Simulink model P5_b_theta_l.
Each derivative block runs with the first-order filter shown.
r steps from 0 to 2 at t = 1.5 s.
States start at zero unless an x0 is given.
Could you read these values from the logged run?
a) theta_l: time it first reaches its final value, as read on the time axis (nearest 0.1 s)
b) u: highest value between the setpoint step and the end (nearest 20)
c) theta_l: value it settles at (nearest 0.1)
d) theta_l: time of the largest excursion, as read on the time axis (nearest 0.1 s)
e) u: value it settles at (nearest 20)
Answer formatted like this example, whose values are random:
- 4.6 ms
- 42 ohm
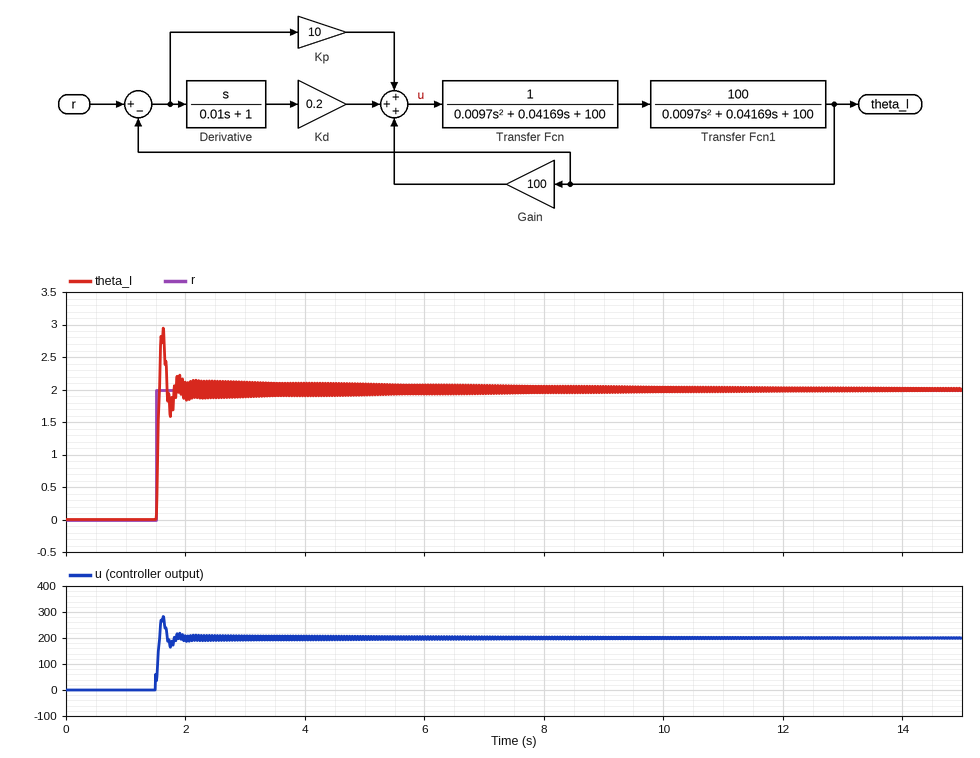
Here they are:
- 1.6 s
- 280
- 2.0
- 1.6 s
- 200
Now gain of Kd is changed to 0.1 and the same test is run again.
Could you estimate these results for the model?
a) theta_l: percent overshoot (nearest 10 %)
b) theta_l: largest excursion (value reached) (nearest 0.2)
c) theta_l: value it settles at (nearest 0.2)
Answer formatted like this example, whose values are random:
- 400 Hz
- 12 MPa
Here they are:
- 60 %
- 3.2
- 2.0
